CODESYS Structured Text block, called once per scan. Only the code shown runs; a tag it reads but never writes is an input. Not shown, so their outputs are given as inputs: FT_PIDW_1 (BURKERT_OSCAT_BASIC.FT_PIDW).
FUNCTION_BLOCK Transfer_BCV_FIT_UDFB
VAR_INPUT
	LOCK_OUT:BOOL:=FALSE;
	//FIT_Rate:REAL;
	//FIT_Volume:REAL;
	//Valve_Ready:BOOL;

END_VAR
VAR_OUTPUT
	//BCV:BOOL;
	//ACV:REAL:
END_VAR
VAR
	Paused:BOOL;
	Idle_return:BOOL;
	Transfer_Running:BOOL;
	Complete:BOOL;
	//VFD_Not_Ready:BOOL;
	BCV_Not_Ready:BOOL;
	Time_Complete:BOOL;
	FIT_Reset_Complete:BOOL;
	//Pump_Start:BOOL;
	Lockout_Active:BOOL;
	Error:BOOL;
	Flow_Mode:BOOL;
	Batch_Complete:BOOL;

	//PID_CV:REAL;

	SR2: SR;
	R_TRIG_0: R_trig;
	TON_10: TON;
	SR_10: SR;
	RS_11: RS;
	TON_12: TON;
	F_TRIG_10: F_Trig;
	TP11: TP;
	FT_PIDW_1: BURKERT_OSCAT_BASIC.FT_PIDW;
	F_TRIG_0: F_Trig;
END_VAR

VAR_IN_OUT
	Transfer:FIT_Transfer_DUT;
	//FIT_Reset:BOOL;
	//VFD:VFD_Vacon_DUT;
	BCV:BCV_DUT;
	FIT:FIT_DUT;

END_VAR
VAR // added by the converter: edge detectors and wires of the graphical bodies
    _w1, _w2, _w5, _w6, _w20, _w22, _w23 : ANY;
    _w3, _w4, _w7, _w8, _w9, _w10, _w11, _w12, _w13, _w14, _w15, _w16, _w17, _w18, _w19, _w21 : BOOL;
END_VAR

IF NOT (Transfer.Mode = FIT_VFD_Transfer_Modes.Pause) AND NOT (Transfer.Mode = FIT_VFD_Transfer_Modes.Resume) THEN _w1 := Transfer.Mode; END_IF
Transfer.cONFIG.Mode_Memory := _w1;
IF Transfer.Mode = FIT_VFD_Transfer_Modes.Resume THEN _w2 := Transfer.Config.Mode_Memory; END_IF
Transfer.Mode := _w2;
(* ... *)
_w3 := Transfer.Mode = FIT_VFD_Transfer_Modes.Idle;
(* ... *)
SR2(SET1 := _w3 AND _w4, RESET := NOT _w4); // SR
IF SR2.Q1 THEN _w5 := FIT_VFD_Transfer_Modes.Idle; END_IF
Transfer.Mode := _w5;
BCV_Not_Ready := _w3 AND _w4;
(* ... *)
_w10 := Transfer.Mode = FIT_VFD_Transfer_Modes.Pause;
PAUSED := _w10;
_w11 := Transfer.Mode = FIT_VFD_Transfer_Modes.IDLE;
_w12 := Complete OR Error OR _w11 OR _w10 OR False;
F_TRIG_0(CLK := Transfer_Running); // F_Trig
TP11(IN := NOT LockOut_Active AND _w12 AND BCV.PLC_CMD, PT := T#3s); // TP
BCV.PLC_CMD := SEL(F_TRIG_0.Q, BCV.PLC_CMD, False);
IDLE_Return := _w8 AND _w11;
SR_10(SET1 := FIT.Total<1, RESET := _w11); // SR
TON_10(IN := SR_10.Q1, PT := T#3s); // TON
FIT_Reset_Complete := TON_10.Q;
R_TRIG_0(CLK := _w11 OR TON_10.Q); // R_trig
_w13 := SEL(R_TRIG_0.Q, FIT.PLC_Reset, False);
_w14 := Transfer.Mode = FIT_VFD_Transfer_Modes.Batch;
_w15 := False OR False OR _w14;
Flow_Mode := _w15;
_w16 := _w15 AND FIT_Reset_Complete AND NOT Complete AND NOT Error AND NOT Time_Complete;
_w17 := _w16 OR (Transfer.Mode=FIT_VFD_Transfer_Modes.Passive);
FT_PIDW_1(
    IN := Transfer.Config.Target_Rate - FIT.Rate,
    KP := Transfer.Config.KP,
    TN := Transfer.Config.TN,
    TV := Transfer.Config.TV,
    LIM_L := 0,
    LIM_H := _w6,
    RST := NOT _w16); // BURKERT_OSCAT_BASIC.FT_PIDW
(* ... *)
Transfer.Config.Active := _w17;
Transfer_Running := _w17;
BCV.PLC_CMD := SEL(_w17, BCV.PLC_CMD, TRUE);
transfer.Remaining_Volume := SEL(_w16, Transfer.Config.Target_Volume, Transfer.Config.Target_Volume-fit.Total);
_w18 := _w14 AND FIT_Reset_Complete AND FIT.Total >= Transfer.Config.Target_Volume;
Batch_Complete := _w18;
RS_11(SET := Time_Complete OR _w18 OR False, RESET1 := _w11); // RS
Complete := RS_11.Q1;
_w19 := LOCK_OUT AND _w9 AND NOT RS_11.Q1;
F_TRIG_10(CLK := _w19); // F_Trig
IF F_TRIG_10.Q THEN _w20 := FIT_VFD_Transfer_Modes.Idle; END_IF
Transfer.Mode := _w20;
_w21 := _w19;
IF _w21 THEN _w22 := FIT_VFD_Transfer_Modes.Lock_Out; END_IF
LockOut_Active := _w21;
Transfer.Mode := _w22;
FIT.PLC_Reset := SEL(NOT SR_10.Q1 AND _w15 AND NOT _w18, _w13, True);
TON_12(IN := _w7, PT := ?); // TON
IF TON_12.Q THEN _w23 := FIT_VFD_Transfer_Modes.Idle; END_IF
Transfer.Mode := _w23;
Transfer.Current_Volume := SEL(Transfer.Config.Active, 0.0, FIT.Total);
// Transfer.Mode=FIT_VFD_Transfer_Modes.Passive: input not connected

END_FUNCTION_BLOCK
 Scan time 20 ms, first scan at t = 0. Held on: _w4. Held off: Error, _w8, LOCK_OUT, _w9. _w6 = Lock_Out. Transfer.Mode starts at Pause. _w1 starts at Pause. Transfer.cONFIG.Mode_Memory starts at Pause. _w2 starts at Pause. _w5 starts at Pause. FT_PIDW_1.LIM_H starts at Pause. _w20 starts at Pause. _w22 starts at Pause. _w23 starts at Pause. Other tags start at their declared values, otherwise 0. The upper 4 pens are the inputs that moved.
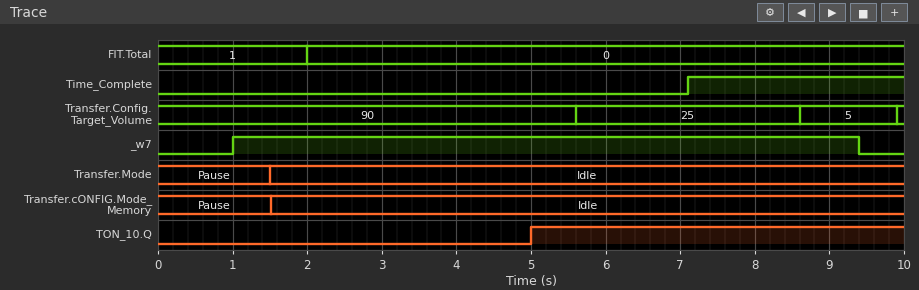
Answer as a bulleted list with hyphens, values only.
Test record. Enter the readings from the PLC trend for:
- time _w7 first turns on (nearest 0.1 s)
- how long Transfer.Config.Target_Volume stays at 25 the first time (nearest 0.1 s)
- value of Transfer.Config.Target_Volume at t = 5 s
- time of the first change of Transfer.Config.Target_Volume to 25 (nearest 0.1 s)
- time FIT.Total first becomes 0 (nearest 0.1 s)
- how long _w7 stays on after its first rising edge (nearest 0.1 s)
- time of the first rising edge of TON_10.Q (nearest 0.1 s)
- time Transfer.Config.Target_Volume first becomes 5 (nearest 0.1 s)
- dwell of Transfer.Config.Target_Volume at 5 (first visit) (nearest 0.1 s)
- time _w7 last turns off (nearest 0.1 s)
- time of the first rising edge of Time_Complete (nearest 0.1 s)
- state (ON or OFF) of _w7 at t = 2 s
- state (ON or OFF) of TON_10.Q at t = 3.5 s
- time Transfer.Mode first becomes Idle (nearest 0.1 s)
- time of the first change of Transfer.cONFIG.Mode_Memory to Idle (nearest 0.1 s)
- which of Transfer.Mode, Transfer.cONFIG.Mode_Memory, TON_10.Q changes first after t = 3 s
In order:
- 1.0 s
- 3.0 s
- 90
- 5.6 s
- 2.0 s
- 8.4 s
- 5.0 s
- 8.6 s
- 1.3 s
- 9.4 s
- 7.1 s
- ON
- OFF
- 1.5 s
- 1.5 s
- TON_10.Q
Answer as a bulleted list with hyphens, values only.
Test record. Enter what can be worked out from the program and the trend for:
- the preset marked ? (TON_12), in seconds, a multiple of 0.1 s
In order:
- 0.5 s
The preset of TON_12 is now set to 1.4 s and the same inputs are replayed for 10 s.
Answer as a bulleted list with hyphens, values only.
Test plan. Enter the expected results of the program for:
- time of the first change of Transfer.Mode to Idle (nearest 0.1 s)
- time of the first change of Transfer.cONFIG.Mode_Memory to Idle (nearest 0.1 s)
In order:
- 2.4 s
- 2.4 s
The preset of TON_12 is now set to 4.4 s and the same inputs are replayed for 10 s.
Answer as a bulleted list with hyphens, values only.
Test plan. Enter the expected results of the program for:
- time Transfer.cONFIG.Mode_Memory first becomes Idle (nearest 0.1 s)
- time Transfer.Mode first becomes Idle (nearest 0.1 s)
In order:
- 5.4 s
- 5.4 s
